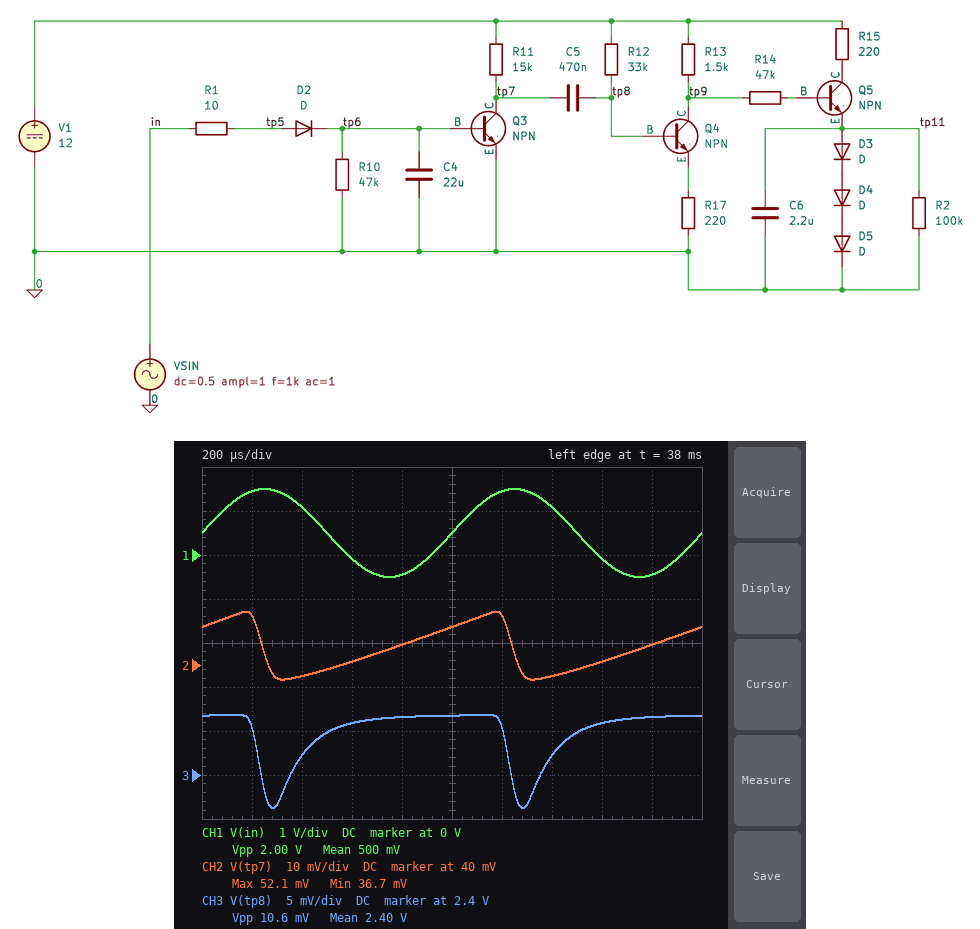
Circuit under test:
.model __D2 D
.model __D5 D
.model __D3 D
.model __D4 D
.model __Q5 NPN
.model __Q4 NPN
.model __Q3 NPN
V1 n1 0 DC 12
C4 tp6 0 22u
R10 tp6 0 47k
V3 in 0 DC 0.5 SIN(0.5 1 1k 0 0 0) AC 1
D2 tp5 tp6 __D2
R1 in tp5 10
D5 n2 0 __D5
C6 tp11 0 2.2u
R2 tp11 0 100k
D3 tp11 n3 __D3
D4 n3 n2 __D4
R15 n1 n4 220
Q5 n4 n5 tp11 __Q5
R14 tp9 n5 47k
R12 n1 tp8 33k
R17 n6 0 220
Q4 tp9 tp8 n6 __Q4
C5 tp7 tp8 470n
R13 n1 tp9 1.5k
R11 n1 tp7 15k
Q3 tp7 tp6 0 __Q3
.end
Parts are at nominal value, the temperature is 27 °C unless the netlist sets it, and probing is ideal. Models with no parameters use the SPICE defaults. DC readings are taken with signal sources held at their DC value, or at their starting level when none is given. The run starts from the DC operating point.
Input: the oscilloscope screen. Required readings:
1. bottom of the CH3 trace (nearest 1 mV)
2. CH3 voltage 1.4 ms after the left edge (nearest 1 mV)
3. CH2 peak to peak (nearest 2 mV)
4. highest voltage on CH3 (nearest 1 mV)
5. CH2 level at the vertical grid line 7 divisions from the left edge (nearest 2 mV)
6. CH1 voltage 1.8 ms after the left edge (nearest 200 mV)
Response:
2.396 V
2.402 V
16 mV
2.407 V
38 mV
-400 mV
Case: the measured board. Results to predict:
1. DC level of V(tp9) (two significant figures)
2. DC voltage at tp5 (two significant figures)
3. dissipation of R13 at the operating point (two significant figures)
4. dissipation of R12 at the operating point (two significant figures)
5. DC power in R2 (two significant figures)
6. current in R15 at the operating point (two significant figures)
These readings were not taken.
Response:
1.7 V
500 mV
71 mW
2.8 mW
10 µW
10 µA
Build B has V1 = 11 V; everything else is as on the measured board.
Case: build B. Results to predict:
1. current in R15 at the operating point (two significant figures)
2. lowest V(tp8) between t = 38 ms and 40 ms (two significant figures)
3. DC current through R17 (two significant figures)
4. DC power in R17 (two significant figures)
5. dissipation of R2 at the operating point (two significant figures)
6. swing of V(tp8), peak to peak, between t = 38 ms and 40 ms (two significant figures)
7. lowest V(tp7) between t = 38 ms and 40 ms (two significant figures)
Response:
8.7 µA
2.3 V
6.6 mA
9.5 mW
7.8 µW
9.7 mV
35 mV
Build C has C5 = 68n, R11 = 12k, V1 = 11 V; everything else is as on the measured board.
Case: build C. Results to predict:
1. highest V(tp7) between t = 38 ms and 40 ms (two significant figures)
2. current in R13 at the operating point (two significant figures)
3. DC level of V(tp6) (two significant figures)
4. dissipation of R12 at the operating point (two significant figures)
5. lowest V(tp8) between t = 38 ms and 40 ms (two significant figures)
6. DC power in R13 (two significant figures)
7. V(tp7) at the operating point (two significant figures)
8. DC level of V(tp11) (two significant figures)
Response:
57 mV
6.3 mA
33 mV
2.3 mW
2.3 V
60 mW
11 V
880 mV
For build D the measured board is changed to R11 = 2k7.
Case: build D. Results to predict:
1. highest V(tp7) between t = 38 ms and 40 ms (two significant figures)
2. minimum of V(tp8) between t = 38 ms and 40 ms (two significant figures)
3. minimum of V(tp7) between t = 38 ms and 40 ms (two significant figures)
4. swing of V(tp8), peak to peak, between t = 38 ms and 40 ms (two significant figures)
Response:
240 mV
2.3 V
81 mV
140 mV
